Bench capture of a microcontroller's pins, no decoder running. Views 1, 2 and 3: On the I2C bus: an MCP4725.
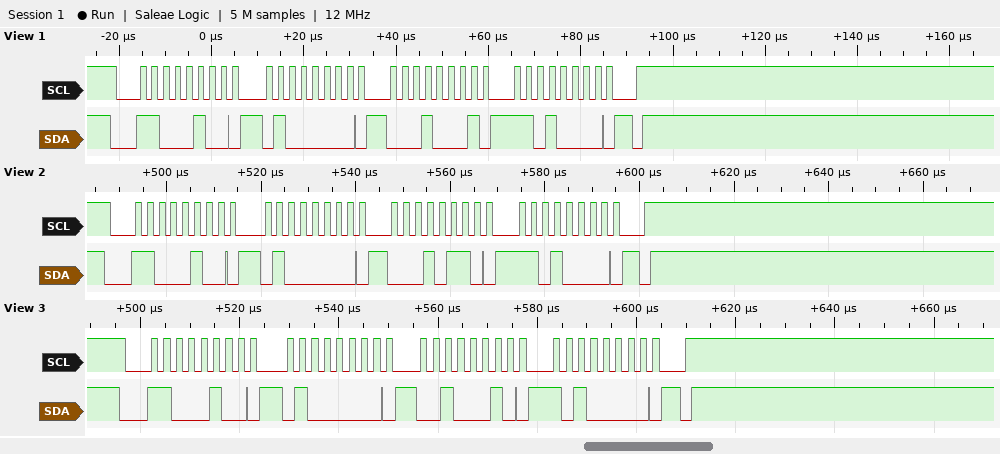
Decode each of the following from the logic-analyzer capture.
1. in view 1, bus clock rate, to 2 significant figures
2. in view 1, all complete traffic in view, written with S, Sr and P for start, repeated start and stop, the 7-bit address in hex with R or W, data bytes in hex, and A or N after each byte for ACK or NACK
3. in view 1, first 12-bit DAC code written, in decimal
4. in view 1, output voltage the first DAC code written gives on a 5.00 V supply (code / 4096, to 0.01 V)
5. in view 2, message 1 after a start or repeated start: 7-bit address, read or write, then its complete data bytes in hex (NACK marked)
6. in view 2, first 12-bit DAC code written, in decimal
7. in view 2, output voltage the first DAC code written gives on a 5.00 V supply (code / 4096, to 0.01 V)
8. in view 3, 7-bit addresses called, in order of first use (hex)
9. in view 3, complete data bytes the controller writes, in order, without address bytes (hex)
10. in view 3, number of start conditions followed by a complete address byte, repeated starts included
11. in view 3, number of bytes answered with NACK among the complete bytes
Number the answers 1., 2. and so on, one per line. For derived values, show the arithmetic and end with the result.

1. 400 kHz
2. S 62W A 40 A 11 A D0 A P
3. 285
4. 285 / 4096 x 5.00 V = 0.35 V
5. 0x62 write: 40 16 D0
6. 365
7. 365 / 4096 x 5.00 V = 0.45 V
8. 0x62
9. 40 22 A0
10. 1
11. 0
